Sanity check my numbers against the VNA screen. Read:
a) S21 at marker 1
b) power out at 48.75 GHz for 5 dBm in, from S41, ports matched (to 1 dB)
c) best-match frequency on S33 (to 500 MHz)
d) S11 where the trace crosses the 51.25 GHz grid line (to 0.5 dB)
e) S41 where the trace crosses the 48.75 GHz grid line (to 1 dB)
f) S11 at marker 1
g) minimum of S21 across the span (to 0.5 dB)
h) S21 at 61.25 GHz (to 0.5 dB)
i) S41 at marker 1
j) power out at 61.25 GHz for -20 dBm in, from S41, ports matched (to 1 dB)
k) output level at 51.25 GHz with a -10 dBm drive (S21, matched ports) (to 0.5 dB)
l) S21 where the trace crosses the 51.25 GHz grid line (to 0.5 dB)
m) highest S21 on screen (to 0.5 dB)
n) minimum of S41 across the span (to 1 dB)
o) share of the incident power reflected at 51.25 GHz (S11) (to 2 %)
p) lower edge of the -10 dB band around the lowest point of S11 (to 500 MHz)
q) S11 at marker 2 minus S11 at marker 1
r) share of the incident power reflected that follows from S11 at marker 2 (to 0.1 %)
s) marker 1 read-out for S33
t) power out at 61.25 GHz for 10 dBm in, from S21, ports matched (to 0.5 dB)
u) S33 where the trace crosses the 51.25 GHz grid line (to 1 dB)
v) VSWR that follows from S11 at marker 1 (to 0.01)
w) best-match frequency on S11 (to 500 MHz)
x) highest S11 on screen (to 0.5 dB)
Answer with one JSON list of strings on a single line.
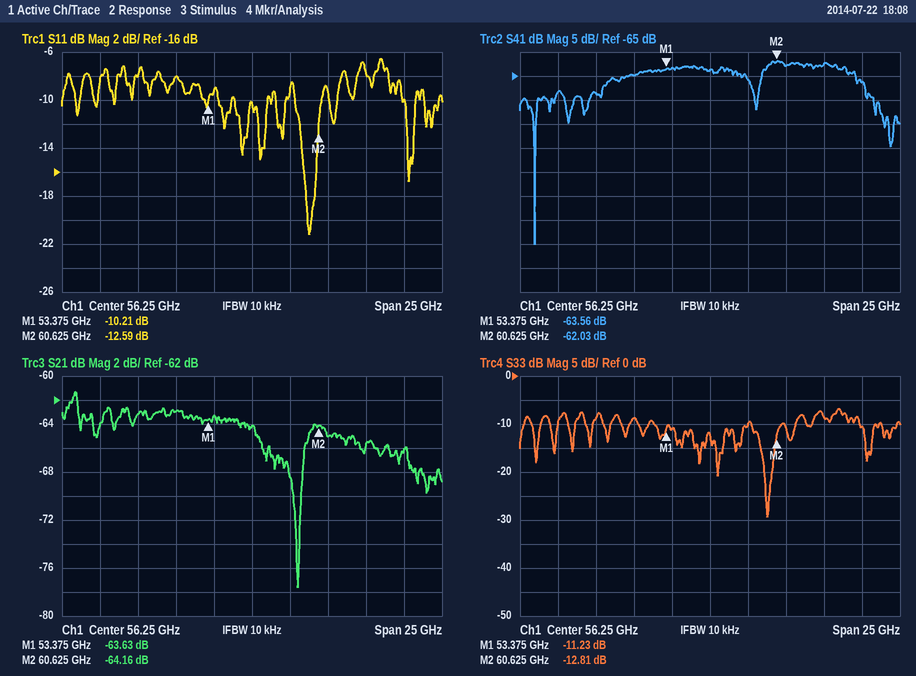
["-63.63 dB", "-64 dBm", "60.0 GHz", "-8.0 dB", "-69 dB", "-10.21 dB", "-77.5 dB", "-65.0 dB", "-63.56 dB", "-83 dBm", "-73.0 dBm", "-63.0 dB", "-61.5 dB", "-100 dB", "16 %", "59.0 GHz", "-2.38 dB", "5.5 %", "-11.23 dB", "-55.0 dBm", "-9 dB", "1.89", "60.0 GHz", "-6.5 dB"]
